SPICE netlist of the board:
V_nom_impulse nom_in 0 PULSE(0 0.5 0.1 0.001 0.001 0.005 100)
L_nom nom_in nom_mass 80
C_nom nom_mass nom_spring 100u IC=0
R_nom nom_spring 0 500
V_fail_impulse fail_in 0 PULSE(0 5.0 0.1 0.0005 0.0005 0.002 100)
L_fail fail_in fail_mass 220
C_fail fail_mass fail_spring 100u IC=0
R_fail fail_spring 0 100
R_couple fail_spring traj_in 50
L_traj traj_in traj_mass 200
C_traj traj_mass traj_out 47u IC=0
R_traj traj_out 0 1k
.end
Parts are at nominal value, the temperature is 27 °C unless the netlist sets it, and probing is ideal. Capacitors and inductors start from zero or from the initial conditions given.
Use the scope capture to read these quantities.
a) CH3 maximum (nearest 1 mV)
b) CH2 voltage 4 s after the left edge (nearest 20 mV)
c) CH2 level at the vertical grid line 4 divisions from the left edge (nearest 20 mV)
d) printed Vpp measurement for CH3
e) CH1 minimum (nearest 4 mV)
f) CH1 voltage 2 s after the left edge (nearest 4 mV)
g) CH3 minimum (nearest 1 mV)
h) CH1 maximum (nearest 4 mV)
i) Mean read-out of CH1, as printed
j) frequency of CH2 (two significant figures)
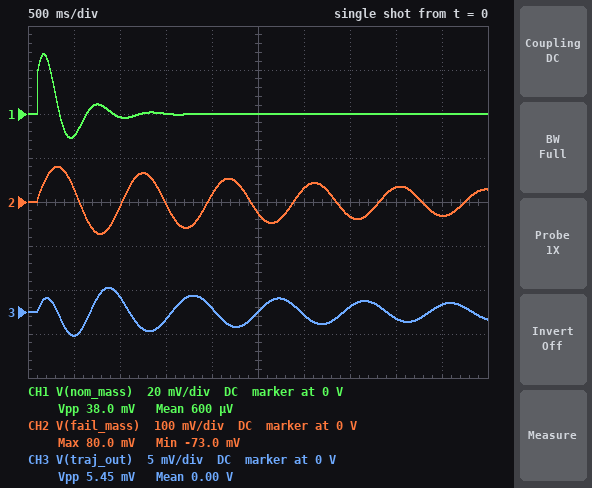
3 mV
40 mV
20 mV
5.45 mV
-12 mV
0 V
-3 mV
28 mV
600 µV
1.1 Hz
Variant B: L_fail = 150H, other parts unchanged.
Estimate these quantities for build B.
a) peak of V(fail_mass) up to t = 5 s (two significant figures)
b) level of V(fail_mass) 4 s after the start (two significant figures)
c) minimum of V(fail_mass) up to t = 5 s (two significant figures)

96 mV
15 mV
-85 mV
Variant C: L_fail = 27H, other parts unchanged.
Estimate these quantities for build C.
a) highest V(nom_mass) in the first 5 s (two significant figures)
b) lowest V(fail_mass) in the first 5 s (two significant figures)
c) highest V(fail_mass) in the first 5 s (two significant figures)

27 mV
-160 mV
210 mV
